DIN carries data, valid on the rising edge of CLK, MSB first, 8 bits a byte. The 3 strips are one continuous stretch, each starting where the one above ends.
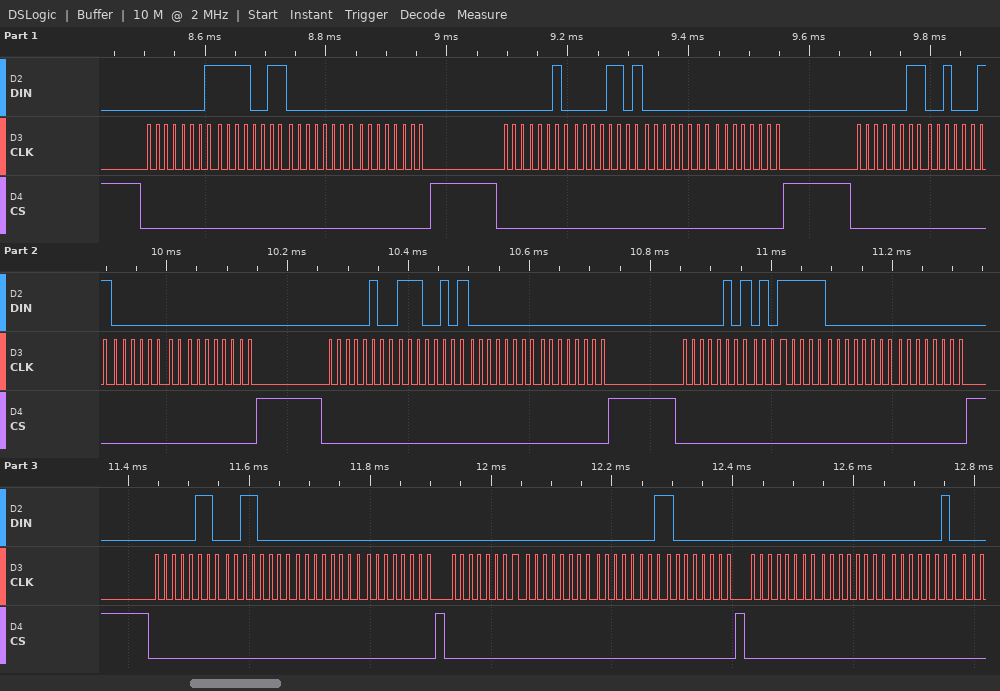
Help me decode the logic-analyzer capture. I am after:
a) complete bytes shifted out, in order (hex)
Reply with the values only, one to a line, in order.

01 F3 00 00 02 0D 00 00 03 23 00 00 04 E5 00 00 05 5F 00 00 06 30 00 00 00 00 01 80 00 00 02
